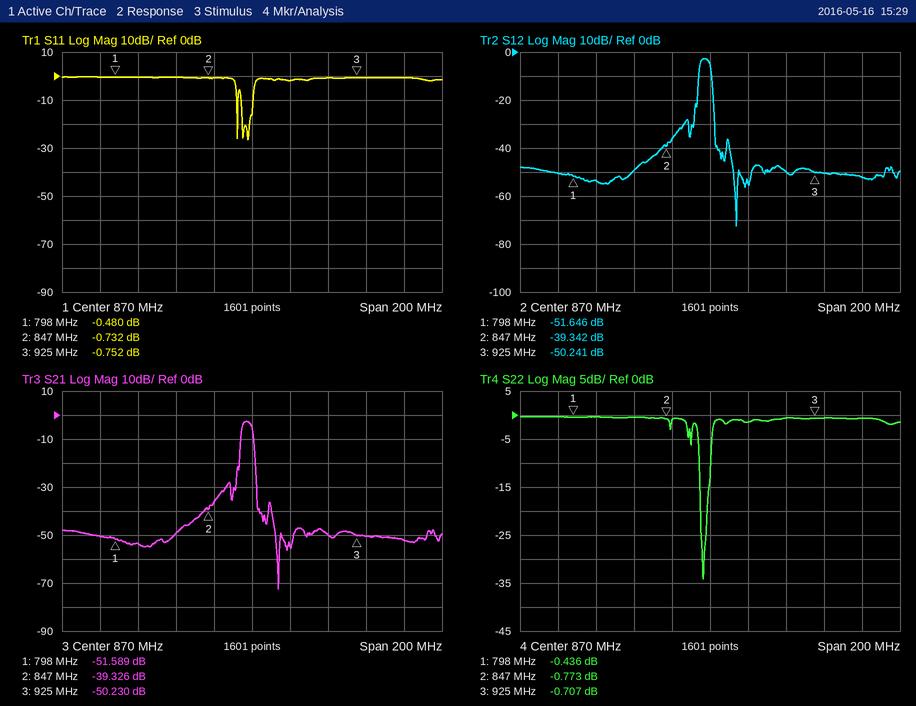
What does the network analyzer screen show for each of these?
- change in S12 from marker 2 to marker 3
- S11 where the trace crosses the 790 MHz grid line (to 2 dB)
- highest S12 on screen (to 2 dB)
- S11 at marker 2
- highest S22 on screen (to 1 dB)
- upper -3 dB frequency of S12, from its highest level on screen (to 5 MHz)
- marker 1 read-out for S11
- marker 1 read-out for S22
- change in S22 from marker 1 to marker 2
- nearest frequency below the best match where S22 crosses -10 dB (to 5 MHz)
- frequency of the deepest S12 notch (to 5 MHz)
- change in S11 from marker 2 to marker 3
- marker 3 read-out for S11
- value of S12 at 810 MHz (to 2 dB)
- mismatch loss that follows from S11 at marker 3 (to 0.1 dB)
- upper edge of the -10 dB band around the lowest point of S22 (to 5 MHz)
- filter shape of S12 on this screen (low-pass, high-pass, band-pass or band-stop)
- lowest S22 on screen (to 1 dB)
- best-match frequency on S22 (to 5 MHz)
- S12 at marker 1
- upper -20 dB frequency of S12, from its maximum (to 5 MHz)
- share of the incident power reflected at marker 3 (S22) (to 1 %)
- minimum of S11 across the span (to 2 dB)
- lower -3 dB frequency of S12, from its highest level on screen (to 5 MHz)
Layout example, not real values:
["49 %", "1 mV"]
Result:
["-10.899 dB", "0 dB", "-2 dB", "-0.732 dB", "0 dB", "870 MHz", "-0.480 dB", "-0.436 dB", "-0.337 dB", "865 MHz", "885 MHz", "-0.020 dB", "-0.752 dB", "-54 dB", "8.0 dB", "870 MHz", "band-pass", "-34 dB", "865 MHz", "-51.646 dB", "870 MHz", "85 %", "-26 dB", "865 MHz"]
